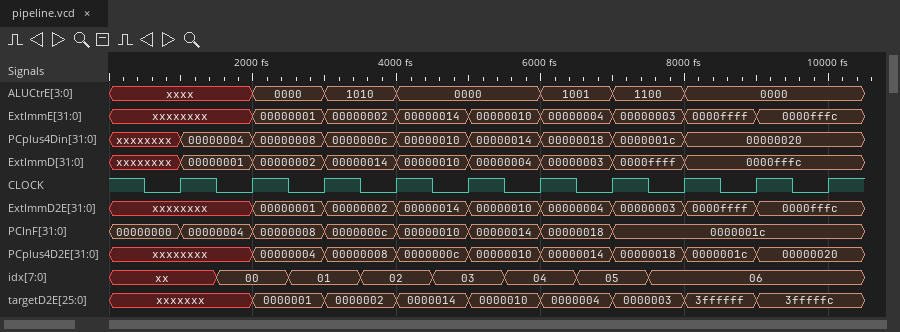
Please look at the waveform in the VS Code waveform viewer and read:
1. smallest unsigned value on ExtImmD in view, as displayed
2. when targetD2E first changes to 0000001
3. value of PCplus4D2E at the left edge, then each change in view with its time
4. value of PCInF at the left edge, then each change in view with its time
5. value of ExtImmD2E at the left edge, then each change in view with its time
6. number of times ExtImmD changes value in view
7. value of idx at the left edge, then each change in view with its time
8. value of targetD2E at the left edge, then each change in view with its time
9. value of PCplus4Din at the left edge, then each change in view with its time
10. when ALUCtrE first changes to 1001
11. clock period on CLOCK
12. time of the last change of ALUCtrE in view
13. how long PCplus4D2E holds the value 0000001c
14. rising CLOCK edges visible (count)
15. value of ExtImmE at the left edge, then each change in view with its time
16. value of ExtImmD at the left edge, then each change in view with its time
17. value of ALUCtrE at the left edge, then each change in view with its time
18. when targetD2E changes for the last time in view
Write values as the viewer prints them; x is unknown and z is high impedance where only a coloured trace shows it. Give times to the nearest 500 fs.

00000001
2000 fs
xxxxxxxx, 00000004 at 2000 fs, 00000008 at 3000 fs, 0000000c at 4000 fs, 00000010 at 5000 fs, 00000014 at 6000 fs, 00000018 at 7000 fs, 0000001c at 8000 fs, 00000020 at 9000 fs
00000000, 00000004 at 1000 fs, 00000008 at 2000 fs, 0000000c at 3000 fs, 00000010 at 4000 fs, 00000014 at 5000 fs, 00000018 at 6000 fs, 0000001c at 7000 fs
xxxxxxxx, 00000001 at 2000 fs, 00000002 at 3000 fs, 00000014 at 4000 fs, 00000010 at 5000 fs, 00000004 at 6000 fs, 00000003 at 7000 fs, 0000ffff at 8000 fs, 0000fffc at 9000 fs
8
xx, 00 at 1500 fs, 01 at 2500 fs, 02 at 3500 fs, 03 at 4500 fs, 04 at 5500 fs, 05 at 6500 fs, 06 at 7500 fs
xxxxxxx, 0000001 at 2000 fs, 0000002 at 3000 fs, 0000014 at 4000 fs, 0000010 at 5000 fs, 0000004 at 6000 fs, 0000003 at 7000 fs, 3ffffff at 8000 fs, 3fffffc at 9000 fs
xxxxxxxx, 00000004 at 1000 fs, 00000008 at 2000 fs, 0000000c at 3000 fs, 00000010 at 4000 fs, 00000014 at 5000 fs, 00000018 at 6000 fs, 0000001c at 7000 fs, 00000020 at 8000 fs
6000 fs
1000 fs
8000 fs
1000 fs
10
xxxxxxxx, 00000001 at 2000 fs, 00000002 at 3000 fs, 00000014 at 4000 fs, 00000010 at 5000 fs, 00000004 at 6000 fs, 00000003 at 7000 fs, 0000ffff at 8000 fs, 0000fffc at 9000 fs
xxxxxxxx, 00000001 at 1000 fs, 00000002 at 2000 fs, 00000014 at 3000 fs, 00000010 at 4000 fs, 00000004 at 5000 fs, 00000003 at 6000 fs, 0000ffff at 7000 fs, 0000fffc at 8000 fs
xxxx, 0000 at 2000 fs, 1010 at 3000 fs, 0000 at 4000 fs, 1001 at 6000 fs, 1100 at 7000 fs, 0000 at 8000 fs
9000 fs
